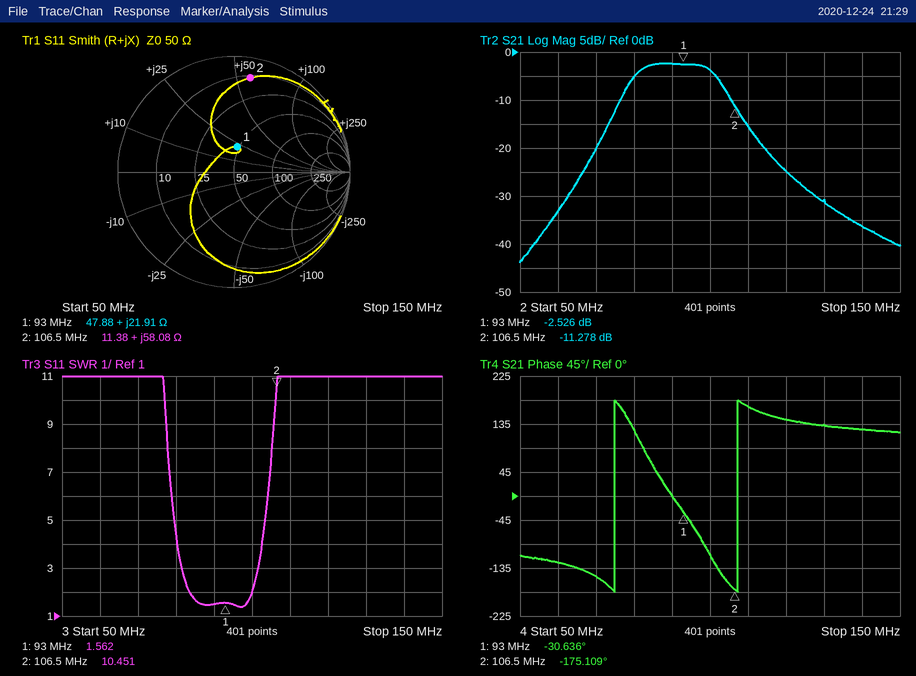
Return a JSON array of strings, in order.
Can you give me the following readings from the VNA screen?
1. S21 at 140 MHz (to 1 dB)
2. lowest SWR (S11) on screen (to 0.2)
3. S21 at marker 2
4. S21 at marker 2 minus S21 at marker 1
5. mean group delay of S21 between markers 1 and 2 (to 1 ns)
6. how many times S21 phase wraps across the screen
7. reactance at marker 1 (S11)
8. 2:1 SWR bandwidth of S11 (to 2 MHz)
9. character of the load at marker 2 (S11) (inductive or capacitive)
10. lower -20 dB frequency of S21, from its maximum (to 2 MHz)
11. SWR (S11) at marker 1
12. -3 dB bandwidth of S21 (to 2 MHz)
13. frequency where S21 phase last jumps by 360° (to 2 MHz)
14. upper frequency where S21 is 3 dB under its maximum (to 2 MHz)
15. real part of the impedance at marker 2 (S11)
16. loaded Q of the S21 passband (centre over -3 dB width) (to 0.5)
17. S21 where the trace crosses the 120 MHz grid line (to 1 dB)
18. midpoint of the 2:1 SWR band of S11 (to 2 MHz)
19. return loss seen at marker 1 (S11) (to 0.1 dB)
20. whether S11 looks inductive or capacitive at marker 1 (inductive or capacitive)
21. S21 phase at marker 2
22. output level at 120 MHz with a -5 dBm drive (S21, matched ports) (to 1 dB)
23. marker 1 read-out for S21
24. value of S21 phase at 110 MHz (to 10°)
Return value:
["-36 dB", "1.4", "-11.278 dB", "-8.752 dB", "30 ns", "2", "+21.91 Ω", "16 MHz", "inductive", "68 MHz", "1.562", "22 MHz", "108 MHz", "102 MHz", "11.38 Ω", "4.0", "-25 dB", "92 MHz", "13.2 dB", "inductive", "-175.109°", "-30 dBm", "-2.526 dB", "170°"]
